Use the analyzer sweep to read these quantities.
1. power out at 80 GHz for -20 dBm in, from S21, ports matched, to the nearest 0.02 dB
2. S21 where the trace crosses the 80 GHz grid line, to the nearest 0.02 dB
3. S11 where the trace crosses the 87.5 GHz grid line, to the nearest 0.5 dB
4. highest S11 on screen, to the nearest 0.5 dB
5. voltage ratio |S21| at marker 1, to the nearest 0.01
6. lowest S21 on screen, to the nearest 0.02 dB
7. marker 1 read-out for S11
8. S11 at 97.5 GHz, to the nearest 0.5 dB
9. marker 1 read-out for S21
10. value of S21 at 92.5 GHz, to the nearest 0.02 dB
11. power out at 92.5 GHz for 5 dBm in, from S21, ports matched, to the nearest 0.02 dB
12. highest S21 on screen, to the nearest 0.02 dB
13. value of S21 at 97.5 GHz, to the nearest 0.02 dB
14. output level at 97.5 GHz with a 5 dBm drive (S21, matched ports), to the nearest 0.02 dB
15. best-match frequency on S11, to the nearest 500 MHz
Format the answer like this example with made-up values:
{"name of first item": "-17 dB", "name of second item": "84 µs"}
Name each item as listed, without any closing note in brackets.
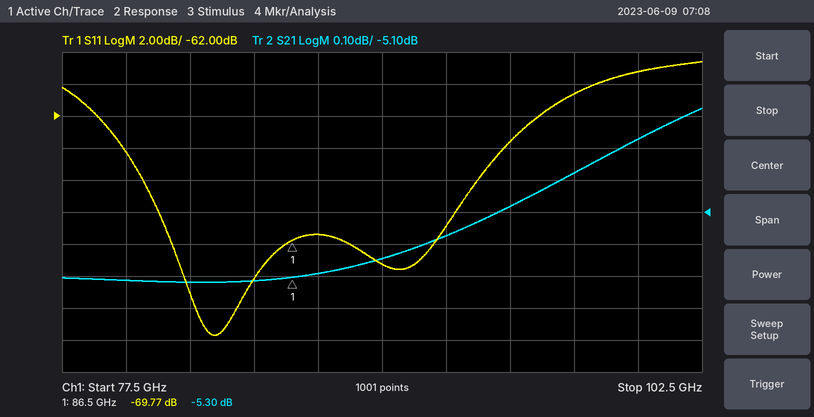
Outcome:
{"power out at 80 GHz for -20 dBm in, from S21, ports matched, to the nearest 0.02 dB": "-25.32 dBm", "S21 where the trace crosses the 80 GHz grid line, to the nearest 0.02 dB": "-5.32 dB", "S11 where the trace crosses the 87.5 GHz grid line, to the nearest 0.5 dB": "-69.5 dB", "highest S11 on screen, to the nearest 0.5 dB": "-58.5 dB", "voltage ratio |S21| at marker 1, to the nearest 0.01": "0.54", "lowest S21 on screen, to the nearest 0.02 dB": "-5.32 dB", "marker 1 read-out for S11": "-69.77 dB", "S11 at 97.5 GHz, to the nearest 0.5 dB": "-60.5 dB", "marker 1 read-out for S21": "-5.30 dB", "value of S21 at 92.5 GHz, to the nearest 0.02 dB": "-5.18 dB", "power out at 92.5 GHz for 5 dBm in, from S21, ports matched, to the nearest 0.02 dB": "-0.18 dBm", "highest S21 on screen, to the nearest 0.02 dB": "-4.78 dB", "value of S21 at 97.5 GHz, to the nearest 0.02 dB": "-4.98 dB", "output level at 97.5 GHz with a 5 dBm drive (S21, matched ports), to the nearest 0.02 dB": "0.02 dBm", "best-match frequency on S11, to the nearest 500 MHz": "83.5 GHz"}
